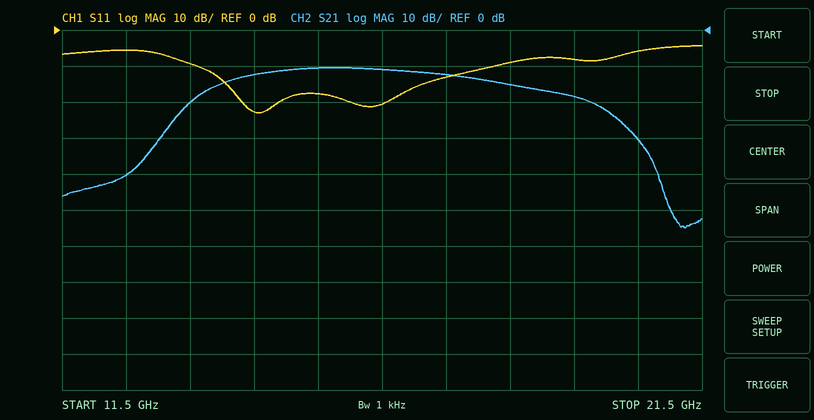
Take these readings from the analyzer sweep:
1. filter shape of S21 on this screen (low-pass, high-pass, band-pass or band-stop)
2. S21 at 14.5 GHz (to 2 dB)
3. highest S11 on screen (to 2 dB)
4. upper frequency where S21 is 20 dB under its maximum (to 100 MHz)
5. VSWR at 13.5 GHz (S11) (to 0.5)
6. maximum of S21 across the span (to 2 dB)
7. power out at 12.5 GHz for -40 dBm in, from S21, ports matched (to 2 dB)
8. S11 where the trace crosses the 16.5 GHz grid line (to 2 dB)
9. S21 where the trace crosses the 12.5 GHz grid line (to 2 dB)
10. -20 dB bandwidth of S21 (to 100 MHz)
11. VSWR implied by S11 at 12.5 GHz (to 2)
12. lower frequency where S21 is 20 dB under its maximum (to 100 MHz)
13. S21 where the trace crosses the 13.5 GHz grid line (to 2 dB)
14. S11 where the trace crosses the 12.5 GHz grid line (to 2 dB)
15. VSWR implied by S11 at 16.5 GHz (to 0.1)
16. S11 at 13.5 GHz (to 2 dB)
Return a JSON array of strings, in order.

["band-pass", "-12 dB", "-4 dB", "20.5 GHz", "2.0", "-10 dB", "-80 dBm", "-20 dB", "-40 dB", "7.5 GHz", "4", "13.0 GHz", "-20 dB", "-6 dB", "1.2", "-10 dB"]
